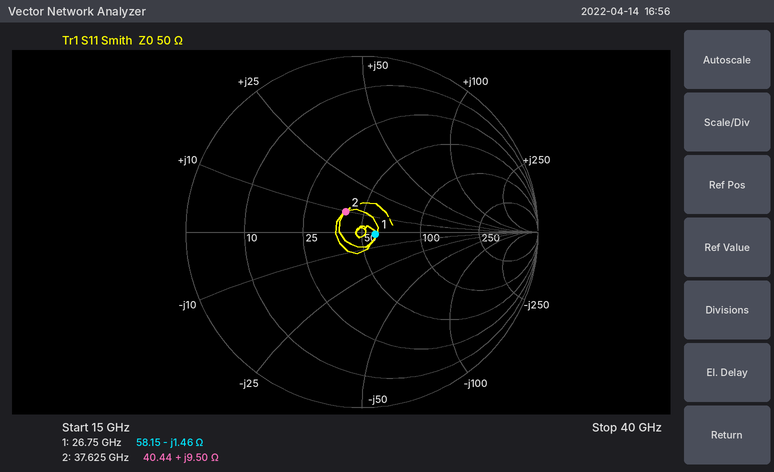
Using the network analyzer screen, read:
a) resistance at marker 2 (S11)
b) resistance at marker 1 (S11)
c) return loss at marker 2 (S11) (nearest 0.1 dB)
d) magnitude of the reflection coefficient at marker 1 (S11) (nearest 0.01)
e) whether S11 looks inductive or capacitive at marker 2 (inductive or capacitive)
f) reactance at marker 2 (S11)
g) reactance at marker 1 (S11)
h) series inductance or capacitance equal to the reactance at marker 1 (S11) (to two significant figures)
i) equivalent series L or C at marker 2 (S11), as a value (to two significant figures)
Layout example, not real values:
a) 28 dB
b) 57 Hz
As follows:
a) 40.44 Ω
b) 58.15 Ω
c) 16.6 dB
d) 0.08
e) inductive
f) +9.50 Ω
g) -1.46 Ω
h) 4.1 pF
i) 40 pH
